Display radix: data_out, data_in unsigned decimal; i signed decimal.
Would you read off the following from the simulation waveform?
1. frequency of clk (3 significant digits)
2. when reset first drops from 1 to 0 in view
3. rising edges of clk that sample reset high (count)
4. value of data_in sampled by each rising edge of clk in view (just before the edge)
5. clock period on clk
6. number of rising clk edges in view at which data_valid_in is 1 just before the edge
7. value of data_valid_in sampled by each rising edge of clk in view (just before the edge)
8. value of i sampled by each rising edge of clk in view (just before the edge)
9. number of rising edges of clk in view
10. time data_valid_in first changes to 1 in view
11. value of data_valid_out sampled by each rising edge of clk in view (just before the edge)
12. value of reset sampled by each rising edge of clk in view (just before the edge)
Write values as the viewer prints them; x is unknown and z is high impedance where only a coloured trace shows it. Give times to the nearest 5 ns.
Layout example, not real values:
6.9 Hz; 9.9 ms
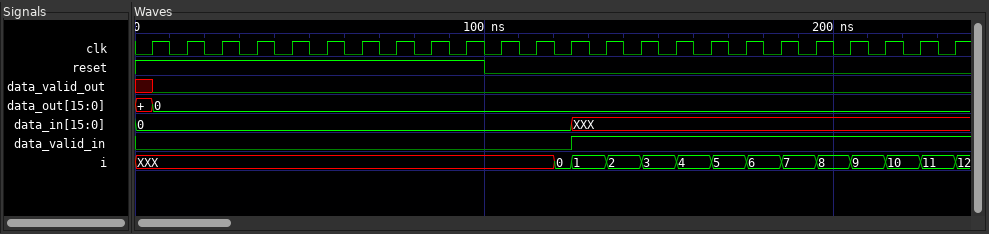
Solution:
100 MHz; 100 ns; 10; 0, 0, 0, 0, 0, 0, 0, 0, 0, 0, 0, 0, 0, XXX, XXX, XXX, XXX, XXX, XXX, XXX, XXX, XXX, XXX, XXX; 10 ns; 11; 0 0 0 0 0 0 0 0 0 0 0 0 0 1 1 1 1 1 1 1 1 1 1 1; XXX, XXX, XXX, XXX, XXX, XXX, XXX, XXX, XXX, XXX, XXX, XXX, 0, 1, 2, 3, 4, 5, 6, 7, 8, 9, 10, 11; 24; 125 ns; x 0 0 0 0 0 0 0 0 0 0 0 0 0 0 0 0 0 0 0 0 0 0 0; 1 1 1 1 1 1 1 1 1 1 0 0 0 0 0 0 0 0 0 0 0 0 0 0
